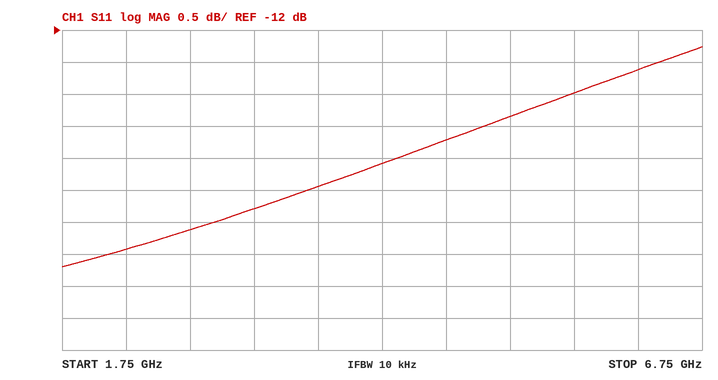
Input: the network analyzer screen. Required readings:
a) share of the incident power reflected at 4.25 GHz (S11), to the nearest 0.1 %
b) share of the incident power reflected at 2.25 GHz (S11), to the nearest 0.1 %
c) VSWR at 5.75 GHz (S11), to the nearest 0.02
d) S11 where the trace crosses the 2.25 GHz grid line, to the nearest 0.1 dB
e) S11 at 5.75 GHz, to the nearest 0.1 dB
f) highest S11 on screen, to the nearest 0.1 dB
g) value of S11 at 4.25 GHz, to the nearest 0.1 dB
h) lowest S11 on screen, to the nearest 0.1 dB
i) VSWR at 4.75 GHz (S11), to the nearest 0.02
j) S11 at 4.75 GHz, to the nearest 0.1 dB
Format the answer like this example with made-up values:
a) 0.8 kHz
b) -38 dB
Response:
a) 3.9 %
b) 2.9 %
c) 1.58
d) -15.4 dB
e) -13.0 dB
f) -12.3 dB
g) -14.1 dB
h) -15.7 dB
i) 1.52
j) -13.7 dB
